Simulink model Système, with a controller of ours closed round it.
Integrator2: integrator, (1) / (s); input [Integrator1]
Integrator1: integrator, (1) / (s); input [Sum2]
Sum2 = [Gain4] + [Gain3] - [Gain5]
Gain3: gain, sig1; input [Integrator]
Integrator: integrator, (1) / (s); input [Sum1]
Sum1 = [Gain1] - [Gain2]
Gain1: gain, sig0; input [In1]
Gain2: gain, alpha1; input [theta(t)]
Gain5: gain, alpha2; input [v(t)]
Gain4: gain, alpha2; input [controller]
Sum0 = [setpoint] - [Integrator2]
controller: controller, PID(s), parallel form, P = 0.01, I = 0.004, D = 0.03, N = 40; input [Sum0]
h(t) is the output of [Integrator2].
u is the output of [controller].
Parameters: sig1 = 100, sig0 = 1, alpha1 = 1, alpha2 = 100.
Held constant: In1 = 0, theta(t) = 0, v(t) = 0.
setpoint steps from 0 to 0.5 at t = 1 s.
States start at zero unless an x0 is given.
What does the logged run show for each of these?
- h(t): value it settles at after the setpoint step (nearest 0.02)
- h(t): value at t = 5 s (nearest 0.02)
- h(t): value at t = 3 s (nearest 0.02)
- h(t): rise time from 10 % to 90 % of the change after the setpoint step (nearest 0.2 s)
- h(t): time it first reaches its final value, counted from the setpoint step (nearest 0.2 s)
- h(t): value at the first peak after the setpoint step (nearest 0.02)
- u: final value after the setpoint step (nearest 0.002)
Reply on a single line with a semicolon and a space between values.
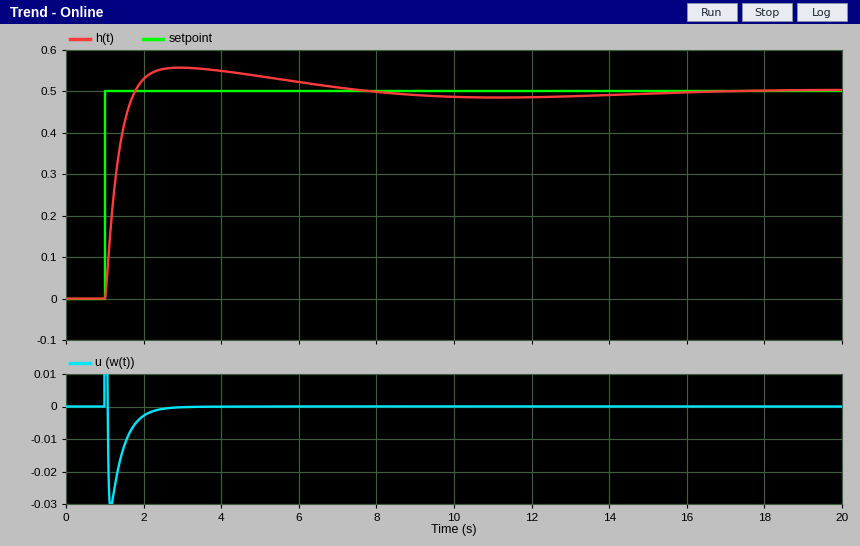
0.50; 0.54; 0.56; 0.6 s; 0.8 s; 0.56; 0.000
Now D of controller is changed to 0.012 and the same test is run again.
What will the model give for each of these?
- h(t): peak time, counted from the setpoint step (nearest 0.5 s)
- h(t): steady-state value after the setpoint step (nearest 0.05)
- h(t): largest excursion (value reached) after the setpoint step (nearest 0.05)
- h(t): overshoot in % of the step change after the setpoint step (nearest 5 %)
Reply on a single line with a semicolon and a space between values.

2.5 s; 0.50; 0.70; 40 %
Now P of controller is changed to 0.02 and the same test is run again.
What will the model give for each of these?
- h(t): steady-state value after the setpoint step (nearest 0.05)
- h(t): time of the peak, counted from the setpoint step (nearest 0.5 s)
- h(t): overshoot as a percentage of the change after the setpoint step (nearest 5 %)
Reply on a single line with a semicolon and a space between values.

0.50; 1.5 s; 15 %
